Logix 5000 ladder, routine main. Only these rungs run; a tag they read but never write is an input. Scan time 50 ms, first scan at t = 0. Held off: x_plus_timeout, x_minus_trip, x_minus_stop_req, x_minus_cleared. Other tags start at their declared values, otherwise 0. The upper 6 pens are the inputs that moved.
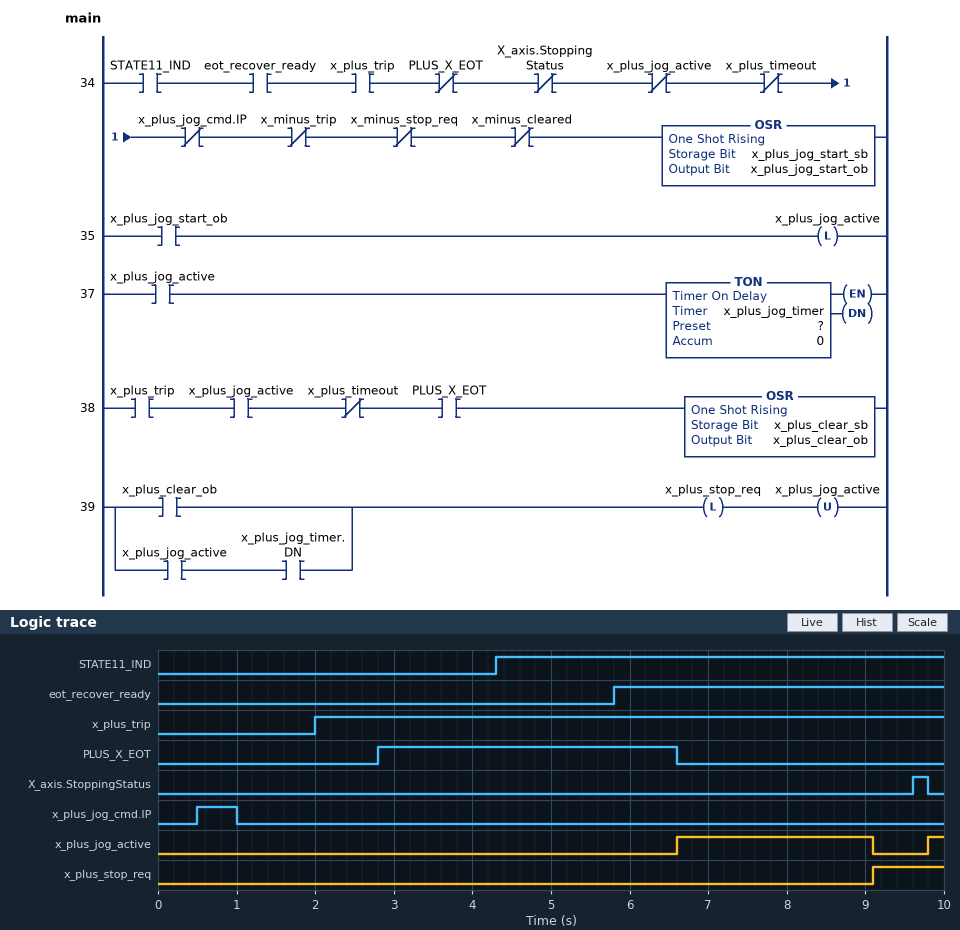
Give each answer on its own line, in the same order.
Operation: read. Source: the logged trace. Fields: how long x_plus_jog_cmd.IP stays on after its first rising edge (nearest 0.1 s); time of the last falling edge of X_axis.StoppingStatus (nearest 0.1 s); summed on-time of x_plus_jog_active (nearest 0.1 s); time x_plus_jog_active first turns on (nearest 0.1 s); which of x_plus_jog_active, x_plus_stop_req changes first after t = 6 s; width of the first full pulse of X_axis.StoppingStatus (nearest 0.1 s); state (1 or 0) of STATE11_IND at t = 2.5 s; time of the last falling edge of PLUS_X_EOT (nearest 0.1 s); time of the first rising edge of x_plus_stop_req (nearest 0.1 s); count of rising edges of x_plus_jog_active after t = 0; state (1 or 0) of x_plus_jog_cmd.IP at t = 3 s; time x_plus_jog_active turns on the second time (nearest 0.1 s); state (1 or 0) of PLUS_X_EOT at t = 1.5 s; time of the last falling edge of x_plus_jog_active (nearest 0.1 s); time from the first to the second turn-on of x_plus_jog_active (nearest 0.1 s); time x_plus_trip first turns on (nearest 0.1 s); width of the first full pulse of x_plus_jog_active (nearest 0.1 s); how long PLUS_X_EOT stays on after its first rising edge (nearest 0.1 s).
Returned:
0.5 s
9.8 s
2.7 s
6.6 s
x_plus_jog_active
0.2 s
0
6.6 s
9.1 s
2
0
9.8 s
0
9.1 s
3.2 s
2.0 s
2.5 s
3.8 s
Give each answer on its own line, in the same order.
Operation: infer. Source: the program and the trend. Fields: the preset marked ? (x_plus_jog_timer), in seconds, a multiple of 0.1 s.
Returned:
2.5 s
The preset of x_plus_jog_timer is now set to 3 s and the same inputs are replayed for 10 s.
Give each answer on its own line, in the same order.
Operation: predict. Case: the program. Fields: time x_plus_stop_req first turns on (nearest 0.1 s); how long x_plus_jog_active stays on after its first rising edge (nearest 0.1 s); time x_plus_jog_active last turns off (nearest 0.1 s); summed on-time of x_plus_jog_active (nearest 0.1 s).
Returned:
9.6 s
3.0 s
9.6 s
3.2 s
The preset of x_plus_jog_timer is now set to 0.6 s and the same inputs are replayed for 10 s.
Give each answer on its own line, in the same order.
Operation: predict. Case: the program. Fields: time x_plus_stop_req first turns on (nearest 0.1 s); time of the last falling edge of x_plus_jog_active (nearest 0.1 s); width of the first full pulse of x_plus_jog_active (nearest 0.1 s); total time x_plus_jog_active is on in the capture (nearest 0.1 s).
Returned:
7.2 s
7.2 s
0.6 s
0.8 s
